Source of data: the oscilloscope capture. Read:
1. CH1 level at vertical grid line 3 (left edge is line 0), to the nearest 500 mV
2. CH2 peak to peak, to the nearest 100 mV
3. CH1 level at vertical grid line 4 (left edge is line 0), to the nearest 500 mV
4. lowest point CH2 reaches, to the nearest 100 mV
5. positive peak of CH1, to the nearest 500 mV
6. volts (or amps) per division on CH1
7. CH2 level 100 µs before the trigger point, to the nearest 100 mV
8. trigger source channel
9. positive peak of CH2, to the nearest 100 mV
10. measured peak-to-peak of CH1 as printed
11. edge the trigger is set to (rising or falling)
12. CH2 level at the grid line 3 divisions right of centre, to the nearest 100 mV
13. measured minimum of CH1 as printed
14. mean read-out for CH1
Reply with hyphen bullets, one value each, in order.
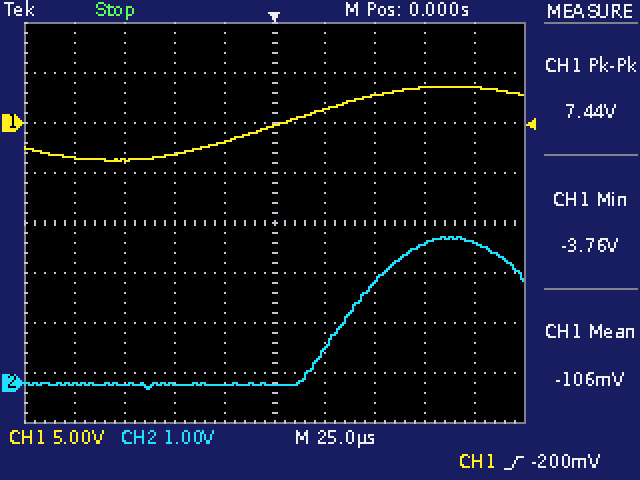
- -3.0 V
- 3.0 V
- -2.0 V
- -100 mV
- 3.5 V
- 5 V
- 0.0 V
- CH1
- 2.9 V
- 7.44 V
- rising
- 2.8 V
- -3.76 V
- -106 mV
